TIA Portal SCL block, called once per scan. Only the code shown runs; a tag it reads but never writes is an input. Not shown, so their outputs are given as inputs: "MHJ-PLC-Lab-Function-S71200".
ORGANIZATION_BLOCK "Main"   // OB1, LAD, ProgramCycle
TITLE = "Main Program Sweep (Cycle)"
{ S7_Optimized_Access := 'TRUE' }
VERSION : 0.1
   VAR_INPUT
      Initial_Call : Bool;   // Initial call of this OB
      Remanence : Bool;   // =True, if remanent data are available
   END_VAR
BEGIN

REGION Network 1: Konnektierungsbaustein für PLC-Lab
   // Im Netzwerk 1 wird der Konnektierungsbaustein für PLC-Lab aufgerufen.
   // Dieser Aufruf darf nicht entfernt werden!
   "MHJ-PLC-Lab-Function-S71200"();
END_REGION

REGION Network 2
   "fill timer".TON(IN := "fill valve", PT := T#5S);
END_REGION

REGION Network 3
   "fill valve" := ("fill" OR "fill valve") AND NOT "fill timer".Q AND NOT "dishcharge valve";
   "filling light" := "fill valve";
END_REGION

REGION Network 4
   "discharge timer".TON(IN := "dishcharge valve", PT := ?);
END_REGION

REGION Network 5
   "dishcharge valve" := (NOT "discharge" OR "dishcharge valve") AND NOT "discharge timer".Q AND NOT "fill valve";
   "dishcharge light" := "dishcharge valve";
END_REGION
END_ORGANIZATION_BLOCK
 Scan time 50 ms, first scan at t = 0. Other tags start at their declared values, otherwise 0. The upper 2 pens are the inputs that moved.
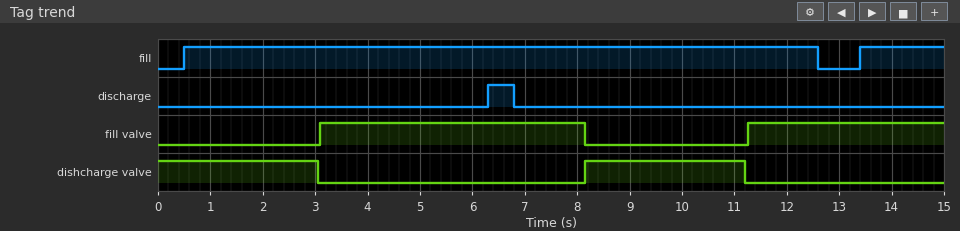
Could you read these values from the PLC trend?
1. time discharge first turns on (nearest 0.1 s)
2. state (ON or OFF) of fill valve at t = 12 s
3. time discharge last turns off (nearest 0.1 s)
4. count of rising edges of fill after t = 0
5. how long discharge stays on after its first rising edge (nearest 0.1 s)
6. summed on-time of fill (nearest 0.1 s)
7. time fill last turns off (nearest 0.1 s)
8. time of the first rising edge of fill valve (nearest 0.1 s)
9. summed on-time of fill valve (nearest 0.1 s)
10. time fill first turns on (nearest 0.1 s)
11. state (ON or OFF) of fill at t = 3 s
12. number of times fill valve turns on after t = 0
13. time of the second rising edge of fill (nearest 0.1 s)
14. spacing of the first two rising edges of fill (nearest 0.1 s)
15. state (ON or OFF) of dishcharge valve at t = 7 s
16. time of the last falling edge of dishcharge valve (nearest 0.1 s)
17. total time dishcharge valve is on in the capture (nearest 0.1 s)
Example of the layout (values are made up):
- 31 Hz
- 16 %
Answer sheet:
- 6.3 s
- ON
- 6.8 s
- 2
- 0.5 s
- 13.7 s
- 12.6 s
- 3.1 s
- 8.8 s
- 0.5 s
- ON
- 2
- 13.4 s
- 12.9 s
- OFF
- 11.2 s
- 6.1 s
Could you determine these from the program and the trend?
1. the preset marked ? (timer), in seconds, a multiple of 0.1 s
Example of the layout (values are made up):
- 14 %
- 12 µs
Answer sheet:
- 3.0 s
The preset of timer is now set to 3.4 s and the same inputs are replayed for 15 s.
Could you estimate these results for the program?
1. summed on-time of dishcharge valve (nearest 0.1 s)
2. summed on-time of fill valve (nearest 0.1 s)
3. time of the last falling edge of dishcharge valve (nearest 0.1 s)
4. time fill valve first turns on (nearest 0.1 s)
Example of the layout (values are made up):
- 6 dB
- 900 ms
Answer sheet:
- 6.9 s
- 8.0 s
- 12.0 s
- 3.5 s
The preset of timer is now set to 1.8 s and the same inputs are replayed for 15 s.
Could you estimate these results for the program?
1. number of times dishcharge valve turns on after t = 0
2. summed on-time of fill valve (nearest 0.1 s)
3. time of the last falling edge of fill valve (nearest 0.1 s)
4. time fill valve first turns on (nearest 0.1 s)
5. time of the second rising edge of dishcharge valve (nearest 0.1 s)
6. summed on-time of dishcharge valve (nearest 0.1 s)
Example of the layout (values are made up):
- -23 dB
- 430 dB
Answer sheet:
- 2
- 10.1 s
- 13.9 s
- 1.9 s
- 13.9 s
- 4.8 s
